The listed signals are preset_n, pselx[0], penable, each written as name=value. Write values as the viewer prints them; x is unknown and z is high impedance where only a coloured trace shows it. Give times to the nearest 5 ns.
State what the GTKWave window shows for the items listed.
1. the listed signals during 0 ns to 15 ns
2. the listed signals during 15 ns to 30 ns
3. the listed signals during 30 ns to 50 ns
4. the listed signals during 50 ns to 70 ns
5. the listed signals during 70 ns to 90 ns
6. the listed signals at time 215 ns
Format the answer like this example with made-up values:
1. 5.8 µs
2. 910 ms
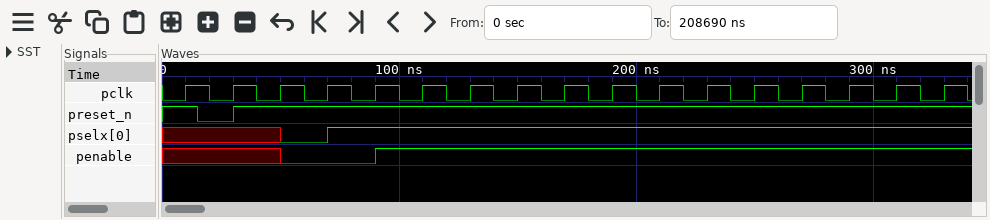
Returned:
1. preset_n=1, pselx[0]=x, penable=x
2. preset_n=0, pselx[0]=x, penable=x
3. preset_n=1, pselx[0]=x, penable=x
4. preset_n=1, pselx[0]=0, penable=0
5. preset_n=1, pselx[0]=1, penable=0
6. preset_n=1, pselx[0]=1, penable=1
